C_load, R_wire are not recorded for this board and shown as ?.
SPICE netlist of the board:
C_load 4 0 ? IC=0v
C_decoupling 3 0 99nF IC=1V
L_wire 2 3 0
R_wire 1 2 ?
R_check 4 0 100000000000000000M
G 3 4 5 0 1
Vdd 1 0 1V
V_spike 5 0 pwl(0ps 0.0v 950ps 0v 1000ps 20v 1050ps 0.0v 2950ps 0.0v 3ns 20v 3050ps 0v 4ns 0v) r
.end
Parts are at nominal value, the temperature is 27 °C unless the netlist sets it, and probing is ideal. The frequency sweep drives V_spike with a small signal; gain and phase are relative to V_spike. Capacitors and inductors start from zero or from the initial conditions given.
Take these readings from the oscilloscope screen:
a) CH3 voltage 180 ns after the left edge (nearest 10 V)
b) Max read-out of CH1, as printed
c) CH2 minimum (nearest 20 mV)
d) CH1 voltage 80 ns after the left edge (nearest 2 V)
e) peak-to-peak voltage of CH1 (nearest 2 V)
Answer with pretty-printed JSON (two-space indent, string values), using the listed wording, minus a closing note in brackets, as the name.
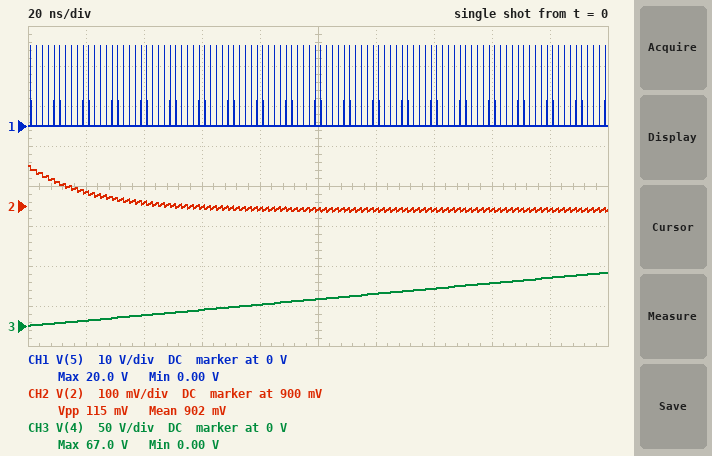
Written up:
{
  "CH3 voltage 180 ns after the left edge": "60 V",
  "Max read-out of CH1, as printed": "20.0 V",
  "CH2 minimum": "880 mV",
  "CH1 voltage 80 ns after the left edge": "0 V",
  "peak-to-peak voltage of CH1": "20 V"
}
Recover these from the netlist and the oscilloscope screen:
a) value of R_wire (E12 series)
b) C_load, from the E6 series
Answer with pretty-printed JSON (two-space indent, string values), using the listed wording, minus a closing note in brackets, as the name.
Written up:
{
  "value of R_wire": "0.22 Ω",
  "C_load, from the E6 series": "1.5 nF"
}
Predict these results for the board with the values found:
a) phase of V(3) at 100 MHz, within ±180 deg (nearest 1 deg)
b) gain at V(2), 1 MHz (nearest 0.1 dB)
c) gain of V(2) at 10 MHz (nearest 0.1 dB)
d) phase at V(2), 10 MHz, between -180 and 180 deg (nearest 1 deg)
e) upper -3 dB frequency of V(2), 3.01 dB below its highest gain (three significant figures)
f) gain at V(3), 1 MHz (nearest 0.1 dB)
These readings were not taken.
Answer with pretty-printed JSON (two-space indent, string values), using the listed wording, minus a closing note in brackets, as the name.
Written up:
{
  "phase of V(3) at 100 MHz, within ±180 deg": "94 deg",
  "gain at V(2), 1 MHz": "-13.2 dB",
  "gain of V(2) at 10 MHz": "-17.7 dB",
  "phase at V(2), 10 MHz, between -180 and 180 deg": "126 deg",
  "upper -3 dB frequency of V(2), 3.01 dB below its highest gain": "7.31 MHz",
  "gain at V(3), 1 MHz": "-13.2 dB"
}
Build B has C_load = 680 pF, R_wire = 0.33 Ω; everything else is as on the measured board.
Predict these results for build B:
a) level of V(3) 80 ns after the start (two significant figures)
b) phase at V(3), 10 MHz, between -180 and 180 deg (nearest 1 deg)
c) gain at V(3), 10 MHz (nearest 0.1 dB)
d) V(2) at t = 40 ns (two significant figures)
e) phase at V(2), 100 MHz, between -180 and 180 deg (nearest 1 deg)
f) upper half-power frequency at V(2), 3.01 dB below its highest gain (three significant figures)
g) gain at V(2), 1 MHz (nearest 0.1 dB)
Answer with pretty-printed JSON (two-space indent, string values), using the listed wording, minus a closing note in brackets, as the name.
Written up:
{
  "level of V(3) 80 ns after the start": "850 mV",
  "phase at V(3), 10 MHz, between -180 and 180 deg": "116 deg",
  "gain at V(3), 10 MHz": "-16.8 dB",
  "V(2) at t = 40 ns": "880 mV",
  "phase at V(2), 100 MHz, between -180 and 180 deg": "93 deg",
  "upper half-power frequency at V(2), 3.01 dB below its highest gain": "4.87 MHz",
  "gain at V(2), 1 MHz": "-9.8 dB"
}
